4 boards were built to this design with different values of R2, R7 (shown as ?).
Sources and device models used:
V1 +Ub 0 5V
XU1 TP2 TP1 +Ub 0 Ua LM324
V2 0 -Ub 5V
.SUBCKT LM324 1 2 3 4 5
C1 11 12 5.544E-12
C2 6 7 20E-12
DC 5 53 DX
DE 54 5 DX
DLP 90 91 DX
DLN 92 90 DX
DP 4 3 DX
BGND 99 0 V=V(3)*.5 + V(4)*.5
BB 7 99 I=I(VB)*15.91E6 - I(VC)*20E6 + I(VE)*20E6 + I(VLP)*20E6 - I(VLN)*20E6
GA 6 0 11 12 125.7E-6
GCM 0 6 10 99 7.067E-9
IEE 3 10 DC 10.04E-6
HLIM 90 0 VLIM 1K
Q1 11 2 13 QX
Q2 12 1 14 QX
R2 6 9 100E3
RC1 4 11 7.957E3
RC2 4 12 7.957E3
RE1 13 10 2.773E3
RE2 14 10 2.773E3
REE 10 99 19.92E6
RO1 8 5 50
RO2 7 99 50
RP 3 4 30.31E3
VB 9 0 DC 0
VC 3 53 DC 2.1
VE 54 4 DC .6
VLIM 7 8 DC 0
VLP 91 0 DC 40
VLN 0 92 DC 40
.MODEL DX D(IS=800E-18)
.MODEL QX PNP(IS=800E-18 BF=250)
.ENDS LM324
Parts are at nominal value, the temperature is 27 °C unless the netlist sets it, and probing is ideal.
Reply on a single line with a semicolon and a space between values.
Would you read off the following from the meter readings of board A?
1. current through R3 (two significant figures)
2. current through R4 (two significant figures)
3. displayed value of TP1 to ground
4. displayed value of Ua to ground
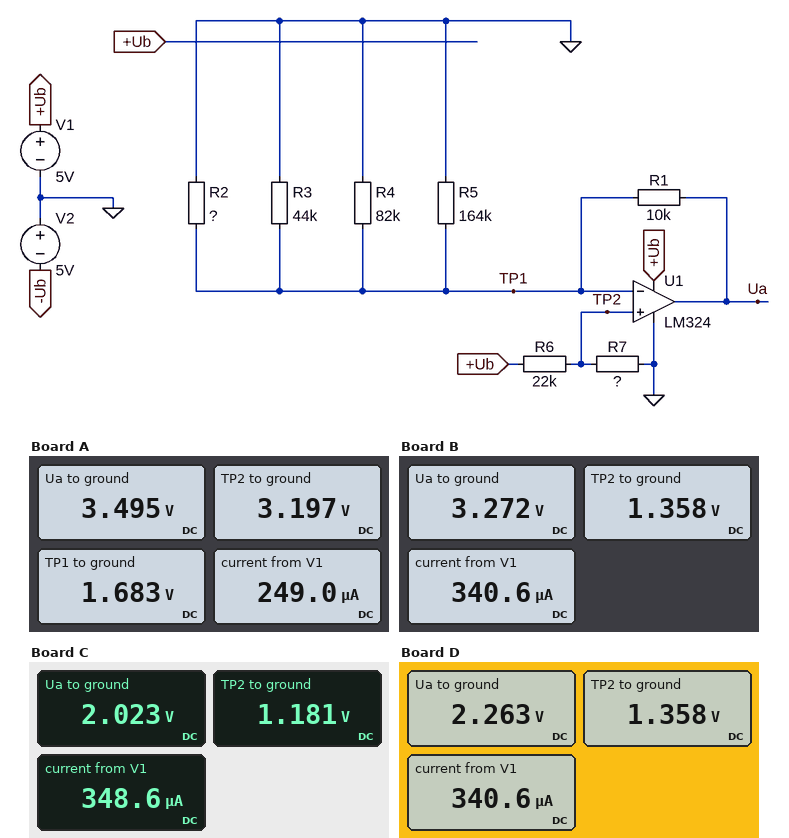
38 µA; 21 µA; 1.683 V; 3.495 V
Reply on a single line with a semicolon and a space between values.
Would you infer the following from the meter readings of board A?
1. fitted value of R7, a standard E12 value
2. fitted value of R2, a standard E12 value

39 kΩ; 15 kΩ
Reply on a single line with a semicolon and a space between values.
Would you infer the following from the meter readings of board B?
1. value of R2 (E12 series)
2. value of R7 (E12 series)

10 kΩ; 8.2 kΩ
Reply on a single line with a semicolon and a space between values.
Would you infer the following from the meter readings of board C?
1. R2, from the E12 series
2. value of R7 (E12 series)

33 kΩ; 6.8 kΩ
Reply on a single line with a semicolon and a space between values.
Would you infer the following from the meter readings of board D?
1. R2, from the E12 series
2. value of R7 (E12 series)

39 kΩ; 8.2 kΩ
